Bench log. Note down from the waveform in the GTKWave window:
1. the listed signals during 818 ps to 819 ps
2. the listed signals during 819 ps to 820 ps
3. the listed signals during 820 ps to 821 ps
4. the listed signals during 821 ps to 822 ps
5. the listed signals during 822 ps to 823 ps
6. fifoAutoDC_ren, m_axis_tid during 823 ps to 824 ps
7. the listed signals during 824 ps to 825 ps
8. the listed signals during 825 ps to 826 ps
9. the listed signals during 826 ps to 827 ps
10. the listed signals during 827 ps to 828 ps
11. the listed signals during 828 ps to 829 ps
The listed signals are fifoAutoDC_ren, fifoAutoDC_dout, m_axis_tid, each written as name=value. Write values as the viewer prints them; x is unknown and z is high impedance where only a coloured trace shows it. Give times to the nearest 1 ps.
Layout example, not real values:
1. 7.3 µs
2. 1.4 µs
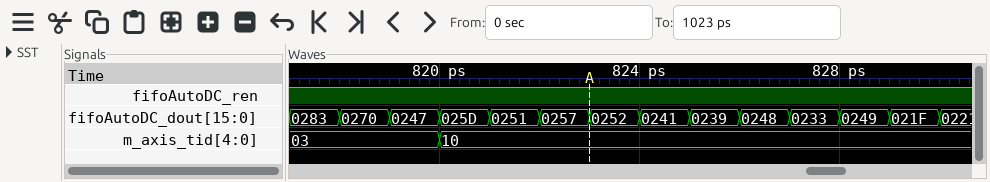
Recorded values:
1. fifoAutoDC_ren=1, fifoAutoDC_dout=0270, m_axis_tid=03
2. fifoAutoDC_ren=1, fifoAutoDC_dout=0247, m_axis_tid=03
3. fifoAutoDC_ren=1, fifoAutoDC_dout=025D, m_axis_tid=10
4. fifoAutoDC_ren=1, fifoAutoDC_dout=0251, m_axis_tid=10
5. fifoAutoDC_ren=1, fifoAutoDC_dout=0257, m_axis_tid=10
6. fifoAutoDC_ren=1, m_axis_tid=10
7. fifoAutoDC_ren=1, fifoAutoDC_dout=0241, m_axis_tid=10
8. fifoAutoDC_ren=1, fifoAutoDC_dout=0239, m_axis_tid=10
9. fifoAutoDC_ren=1, fifoAutoDC_dout=0248, m_axis_tid=10
10. fifoAutoDC_ren=1, fifoAutoDC_dout=0233, m_axis_tid=10
11. fifoAutoDC_ren=1, fifoAutoDC_dout=0249, m_axis_tid=10
